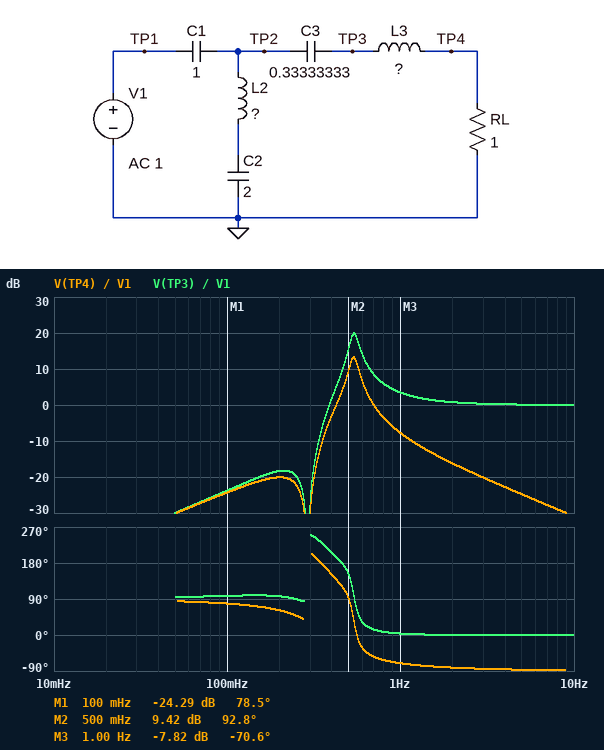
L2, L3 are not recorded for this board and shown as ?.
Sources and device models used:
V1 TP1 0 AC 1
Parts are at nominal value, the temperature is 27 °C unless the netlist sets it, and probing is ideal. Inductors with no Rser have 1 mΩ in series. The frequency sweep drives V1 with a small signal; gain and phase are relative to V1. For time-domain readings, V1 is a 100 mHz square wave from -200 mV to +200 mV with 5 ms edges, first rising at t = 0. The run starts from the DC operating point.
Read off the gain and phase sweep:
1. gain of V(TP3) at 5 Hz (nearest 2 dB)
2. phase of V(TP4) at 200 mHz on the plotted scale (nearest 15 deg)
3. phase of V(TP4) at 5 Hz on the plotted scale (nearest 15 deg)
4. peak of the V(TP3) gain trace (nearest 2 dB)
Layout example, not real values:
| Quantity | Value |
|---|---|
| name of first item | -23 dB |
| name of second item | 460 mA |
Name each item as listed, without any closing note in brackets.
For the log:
| Quantity | Value |
|---|---|
| gain of V(TP3) at 5 Hz | 0 dB |
| phase of V(TP4) at 200 mHz on the plotted scale | 60 deg |
| phase of V(TP4) at 5 Hz on the plotted scale | -90 deg |
| peak of the V(TP3) gain trace | 20 dB |
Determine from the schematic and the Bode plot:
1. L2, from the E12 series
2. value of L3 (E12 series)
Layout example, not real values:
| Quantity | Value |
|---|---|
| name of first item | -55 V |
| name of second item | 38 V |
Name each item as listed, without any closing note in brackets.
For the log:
| Quantity | Value |
|---|---|
| L2, from the E12 series | 150 mH |
| value of L3 | 560 mH |
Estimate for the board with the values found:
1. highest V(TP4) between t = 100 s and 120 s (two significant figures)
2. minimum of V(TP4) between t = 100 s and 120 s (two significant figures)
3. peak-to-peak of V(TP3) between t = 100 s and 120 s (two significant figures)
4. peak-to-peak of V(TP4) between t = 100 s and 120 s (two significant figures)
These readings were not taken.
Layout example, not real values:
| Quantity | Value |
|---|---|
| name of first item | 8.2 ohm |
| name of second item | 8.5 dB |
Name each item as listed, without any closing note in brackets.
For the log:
| Quantity | Value |
|---|---|
| highest V(TP4) between t = 100 s and 120 s | 190 mV |
| minimum of V(TP4) between t = 100 s and 120 s | -190 mV |
| peak-to-peak of V(TP3) between t = 100 s and 120 s | 790 mV |
| peak-to-peak of V(TP4) between t = 100 s and 120 s | 380 mV |
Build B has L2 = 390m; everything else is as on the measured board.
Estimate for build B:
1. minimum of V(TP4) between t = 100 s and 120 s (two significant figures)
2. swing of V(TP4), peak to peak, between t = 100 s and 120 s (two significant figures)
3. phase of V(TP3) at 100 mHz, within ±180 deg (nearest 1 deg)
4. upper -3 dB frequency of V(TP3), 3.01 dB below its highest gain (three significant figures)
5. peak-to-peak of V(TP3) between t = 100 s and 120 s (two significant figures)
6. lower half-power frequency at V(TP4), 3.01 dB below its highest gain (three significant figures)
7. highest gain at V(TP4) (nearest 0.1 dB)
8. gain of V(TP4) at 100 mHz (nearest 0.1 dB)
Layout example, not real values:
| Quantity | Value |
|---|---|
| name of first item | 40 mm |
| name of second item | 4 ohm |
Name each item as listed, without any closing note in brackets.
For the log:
| Quantity | Value |
|---|---|
| minimum of V(TP4) between t = 100 s and 120 s | -240 mV |
| swing of V(TP4), peak to peak, between t = 100 s and 120 s | 470 mV |
| phase of V(TP3) at 100 mHz, within ±180 deg | 98 deg |
| upper -3 dB frequency of V(TP3), 3.01 dB below its highest gain | 582 mHz |
| peak-to-peak of V(TP3) between t = 100 s and 120 s | 880 mV |
| lower half-power frequency at V(TP4), 3.01 dB below its highest gain | 268 mHz |
| highest gain at V(TP4) | 6.6 dB |
| gain of V(TP4) at 100 mHz | -25.7 dB |
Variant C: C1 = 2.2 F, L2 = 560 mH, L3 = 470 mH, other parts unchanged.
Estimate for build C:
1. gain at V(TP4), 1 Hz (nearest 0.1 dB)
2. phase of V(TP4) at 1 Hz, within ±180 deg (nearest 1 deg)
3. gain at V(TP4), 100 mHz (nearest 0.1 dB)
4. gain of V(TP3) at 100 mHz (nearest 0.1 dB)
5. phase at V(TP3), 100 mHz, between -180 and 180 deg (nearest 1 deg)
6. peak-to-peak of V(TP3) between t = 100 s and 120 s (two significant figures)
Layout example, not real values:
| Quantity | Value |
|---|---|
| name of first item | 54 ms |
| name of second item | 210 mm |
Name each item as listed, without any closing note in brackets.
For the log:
| Quantity | Value |
|---|---|
| gain at V(TP4), 1 Hz | -8.1 dB |
| phase of V(TP4) at 1 Hz, within ±180 deg | -67 deg |
| gain at V(TP4), 100 mHz | -22.1 dB |
| gain of V(TP3) at 100 mHz | -21.8 dB |
| phase at V(TP3), 100 mHz, between -180 and 180 deg | 95 deg |
| peak-to-peak of V(TP3) between t = 100 s and 120 s | 810 mV |
